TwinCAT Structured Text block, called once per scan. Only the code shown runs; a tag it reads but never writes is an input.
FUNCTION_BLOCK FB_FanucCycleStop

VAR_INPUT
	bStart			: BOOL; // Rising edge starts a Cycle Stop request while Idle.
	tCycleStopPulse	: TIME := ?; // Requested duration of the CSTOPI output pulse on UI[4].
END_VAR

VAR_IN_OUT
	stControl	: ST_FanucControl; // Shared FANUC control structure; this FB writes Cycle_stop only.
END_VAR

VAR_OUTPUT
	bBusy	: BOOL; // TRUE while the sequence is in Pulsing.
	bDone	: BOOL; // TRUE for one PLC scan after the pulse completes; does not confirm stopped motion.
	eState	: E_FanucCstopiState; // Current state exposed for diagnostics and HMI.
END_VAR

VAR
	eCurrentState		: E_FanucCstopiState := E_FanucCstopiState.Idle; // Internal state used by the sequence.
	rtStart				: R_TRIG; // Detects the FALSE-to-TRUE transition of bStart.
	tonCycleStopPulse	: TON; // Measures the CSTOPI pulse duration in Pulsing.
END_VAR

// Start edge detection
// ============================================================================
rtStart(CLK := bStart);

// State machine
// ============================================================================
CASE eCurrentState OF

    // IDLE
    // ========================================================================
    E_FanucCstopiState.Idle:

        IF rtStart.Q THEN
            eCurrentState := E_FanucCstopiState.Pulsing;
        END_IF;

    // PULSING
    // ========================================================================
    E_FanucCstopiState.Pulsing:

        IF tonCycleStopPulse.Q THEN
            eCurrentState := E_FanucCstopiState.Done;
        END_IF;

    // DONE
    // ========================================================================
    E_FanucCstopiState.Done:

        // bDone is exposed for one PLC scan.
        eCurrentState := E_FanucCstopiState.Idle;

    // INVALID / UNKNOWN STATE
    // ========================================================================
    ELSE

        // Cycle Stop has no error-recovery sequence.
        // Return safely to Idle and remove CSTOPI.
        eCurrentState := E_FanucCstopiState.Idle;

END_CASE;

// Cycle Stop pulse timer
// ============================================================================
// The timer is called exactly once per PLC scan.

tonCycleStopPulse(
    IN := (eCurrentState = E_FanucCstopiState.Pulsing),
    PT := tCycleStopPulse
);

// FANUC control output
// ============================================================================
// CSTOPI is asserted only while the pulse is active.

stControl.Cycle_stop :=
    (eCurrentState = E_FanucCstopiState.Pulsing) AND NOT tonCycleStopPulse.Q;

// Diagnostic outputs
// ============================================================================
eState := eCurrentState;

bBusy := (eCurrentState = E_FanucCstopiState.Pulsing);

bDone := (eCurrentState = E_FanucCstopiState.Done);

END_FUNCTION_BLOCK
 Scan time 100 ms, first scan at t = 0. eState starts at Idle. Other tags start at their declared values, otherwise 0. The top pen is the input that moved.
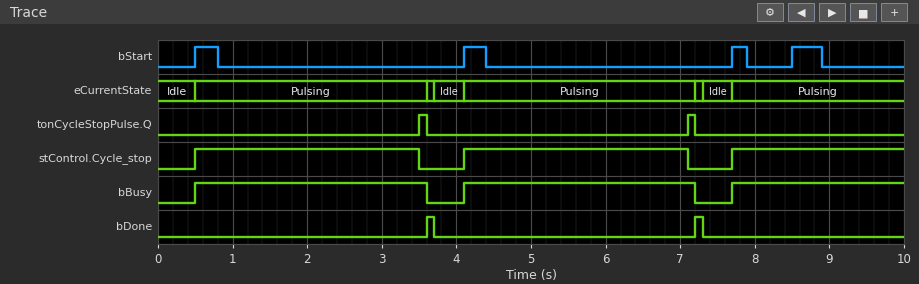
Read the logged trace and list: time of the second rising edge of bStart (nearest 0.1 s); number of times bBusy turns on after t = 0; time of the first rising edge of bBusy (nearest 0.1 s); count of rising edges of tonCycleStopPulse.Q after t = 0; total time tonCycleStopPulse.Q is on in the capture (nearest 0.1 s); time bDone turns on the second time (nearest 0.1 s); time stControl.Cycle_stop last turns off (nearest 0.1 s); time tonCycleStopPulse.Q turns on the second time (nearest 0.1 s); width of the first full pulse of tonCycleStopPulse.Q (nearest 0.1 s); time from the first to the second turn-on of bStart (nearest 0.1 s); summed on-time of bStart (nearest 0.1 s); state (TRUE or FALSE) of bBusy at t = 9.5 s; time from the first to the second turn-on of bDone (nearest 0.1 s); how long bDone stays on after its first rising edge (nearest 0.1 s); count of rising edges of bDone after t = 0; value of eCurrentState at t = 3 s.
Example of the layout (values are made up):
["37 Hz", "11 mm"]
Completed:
["4.1 s", "3", "0.5 s", "2", "0.2 s", "7.2 s", "7.1 s", "7.1 s", "0.1 s", "3.6 s", "1.2 s", "TRUE", "3.6 s", "0.1 s", "2", "Pulsing"]
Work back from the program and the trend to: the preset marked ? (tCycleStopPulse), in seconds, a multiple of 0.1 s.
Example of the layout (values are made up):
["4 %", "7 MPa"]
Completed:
["3.0 s"]
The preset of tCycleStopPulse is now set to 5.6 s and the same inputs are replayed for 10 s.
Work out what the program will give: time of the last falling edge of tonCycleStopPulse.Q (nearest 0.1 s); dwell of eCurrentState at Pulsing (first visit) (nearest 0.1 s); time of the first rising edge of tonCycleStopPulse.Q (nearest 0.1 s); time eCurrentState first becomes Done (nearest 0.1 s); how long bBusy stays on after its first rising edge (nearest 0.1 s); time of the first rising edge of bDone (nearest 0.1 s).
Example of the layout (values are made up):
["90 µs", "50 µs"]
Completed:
["6.2 s", "5.7 s", "6.1 s", "6.2 s", "5.7 s", "6.2 s"]
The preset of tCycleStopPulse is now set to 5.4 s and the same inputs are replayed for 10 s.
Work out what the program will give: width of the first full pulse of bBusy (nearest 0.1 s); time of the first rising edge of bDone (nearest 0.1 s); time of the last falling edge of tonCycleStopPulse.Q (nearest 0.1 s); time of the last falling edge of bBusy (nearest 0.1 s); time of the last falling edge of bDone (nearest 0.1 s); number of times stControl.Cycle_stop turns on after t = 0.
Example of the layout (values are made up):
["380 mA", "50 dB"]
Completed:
["5.5 s", "6.0 s", "6.0 s", "6.0 s", "6.1 s", "2"]
